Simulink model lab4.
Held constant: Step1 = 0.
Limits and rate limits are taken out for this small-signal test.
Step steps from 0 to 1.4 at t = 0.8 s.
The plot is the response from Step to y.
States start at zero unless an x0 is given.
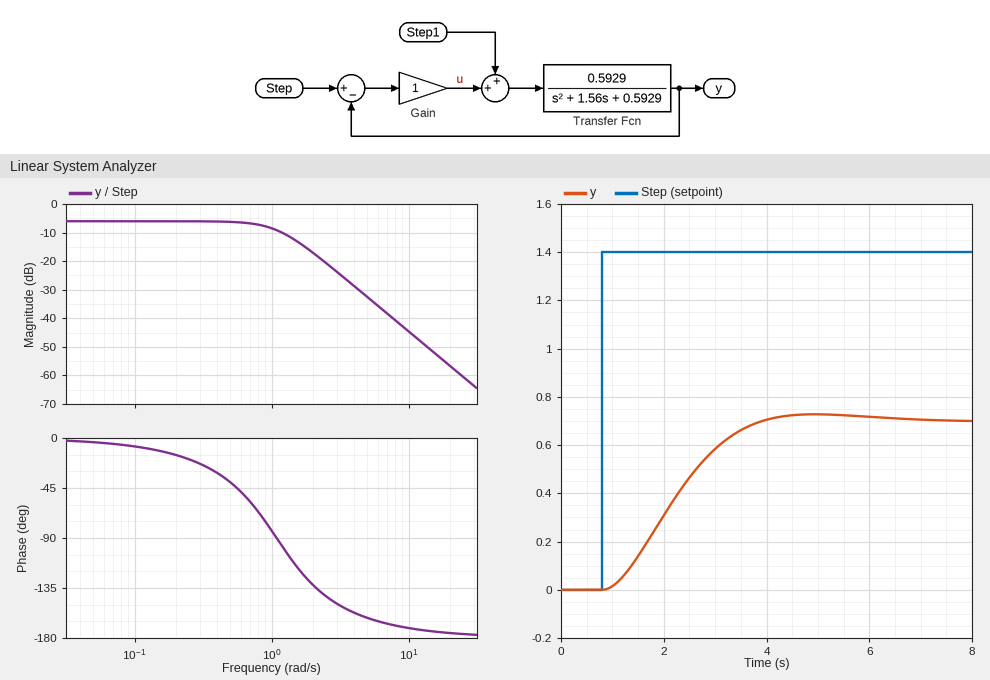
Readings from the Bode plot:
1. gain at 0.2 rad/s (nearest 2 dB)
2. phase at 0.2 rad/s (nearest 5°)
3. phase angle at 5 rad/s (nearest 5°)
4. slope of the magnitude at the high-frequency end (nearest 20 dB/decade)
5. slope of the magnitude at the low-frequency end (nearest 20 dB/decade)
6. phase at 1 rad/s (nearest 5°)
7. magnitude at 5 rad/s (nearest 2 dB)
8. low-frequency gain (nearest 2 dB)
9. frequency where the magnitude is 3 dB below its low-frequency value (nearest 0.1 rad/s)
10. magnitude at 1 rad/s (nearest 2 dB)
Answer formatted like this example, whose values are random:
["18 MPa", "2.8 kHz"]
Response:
["-6 dB", "-15°", "-160°", "-40 dB/decade", "0 dB/decade", "-85°", "-32 dB", "-6 dB", "1.1 rad/s", "-8 dB"]
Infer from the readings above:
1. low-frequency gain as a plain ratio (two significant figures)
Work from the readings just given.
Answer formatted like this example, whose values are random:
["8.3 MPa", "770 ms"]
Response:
["0.50"]
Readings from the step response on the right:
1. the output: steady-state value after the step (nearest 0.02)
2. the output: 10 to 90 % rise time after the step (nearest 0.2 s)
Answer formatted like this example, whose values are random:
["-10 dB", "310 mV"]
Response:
["0.70", "2.0 s"]
